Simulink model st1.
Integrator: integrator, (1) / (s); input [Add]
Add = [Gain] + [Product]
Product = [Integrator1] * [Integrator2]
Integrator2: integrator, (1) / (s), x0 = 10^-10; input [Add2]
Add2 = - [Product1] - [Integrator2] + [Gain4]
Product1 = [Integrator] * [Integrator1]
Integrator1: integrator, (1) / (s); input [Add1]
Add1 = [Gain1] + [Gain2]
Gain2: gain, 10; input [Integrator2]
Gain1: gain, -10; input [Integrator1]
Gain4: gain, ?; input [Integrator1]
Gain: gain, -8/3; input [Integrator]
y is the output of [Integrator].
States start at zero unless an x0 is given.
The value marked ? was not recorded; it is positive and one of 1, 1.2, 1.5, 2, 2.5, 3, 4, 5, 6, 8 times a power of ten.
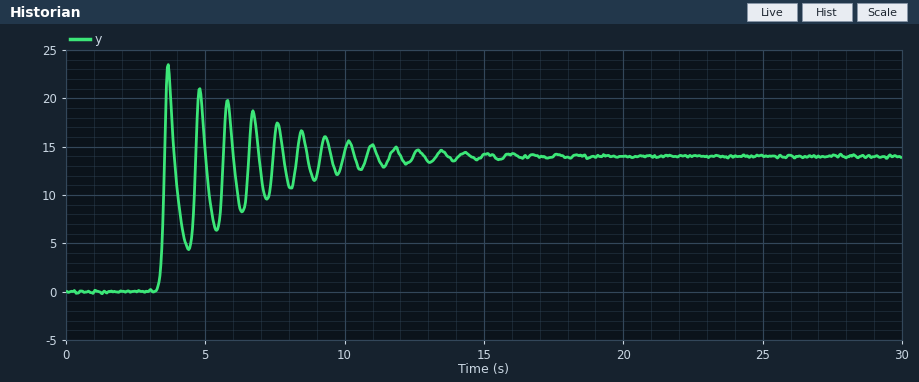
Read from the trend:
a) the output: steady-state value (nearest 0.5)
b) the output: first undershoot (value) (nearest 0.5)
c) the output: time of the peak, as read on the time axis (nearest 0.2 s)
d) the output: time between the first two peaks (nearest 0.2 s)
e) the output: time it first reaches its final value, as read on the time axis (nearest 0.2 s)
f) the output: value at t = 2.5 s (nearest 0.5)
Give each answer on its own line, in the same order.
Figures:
14.0
4.5
3.6 s
1.2 s
3.6 s
0.0
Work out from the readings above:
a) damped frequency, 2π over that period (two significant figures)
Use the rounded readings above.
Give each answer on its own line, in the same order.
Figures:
5.2 rad/s
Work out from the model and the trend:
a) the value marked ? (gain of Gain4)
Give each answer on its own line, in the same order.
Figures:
15
